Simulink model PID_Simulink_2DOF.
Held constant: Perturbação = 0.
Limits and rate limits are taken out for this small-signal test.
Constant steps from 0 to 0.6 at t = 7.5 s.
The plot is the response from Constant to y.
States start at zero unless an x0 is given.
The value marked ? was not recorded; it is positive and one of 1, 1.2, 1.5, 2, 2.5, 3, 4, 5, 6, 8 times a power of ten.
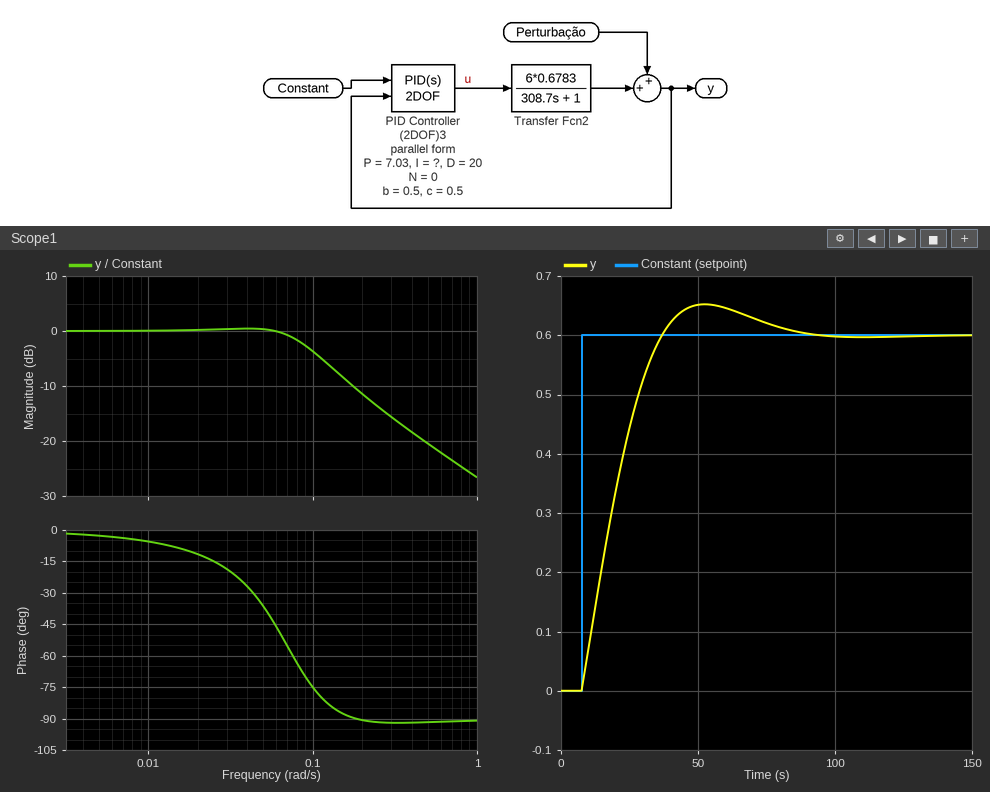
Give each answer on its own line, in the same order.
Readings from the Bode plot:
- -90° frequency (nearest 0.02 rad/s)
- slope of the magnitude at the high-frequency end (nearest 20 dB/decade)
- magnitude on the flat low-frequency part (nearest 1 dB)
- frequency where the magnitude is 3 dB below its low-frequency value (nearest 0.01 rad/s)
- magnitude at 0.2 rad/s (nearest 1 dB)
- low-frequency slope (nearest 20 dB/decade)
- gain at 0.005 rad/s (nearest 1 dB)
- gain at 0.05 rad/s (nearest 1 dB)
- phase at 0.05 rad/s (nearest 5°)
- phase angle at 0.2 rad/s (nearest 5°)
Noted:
0.18 rad/s
-20 dB/decade
0 dB
0.09 rad/s
-11 dB
0 dB/decade
0 dB
0 dB
-35°
-90°
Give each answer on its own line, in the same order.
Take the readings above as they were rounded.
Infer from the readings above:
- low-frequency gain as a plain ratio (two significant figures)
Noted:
1.0
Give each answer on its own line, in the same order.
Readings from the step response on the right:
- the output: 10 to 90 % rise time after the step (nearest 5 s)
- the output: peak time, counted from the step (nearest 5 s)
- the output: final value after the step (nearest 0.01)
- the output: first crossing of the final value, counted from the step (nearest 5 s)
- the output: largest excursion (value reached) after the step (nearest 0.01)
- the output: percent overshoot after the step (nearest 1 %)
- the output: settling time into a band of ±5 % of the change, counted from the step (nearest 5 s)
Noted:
20 s
45 s
0.60
30 s
0.65
9 %
60 s
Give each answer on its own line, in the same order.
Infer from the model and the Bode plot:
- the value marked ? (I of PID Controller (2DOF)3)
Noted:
0.4
